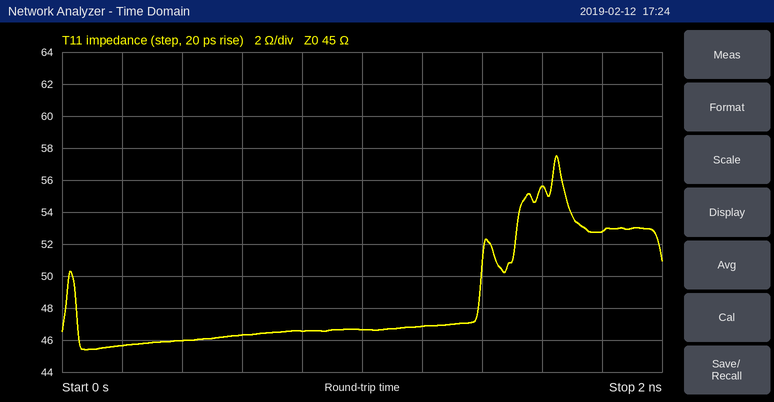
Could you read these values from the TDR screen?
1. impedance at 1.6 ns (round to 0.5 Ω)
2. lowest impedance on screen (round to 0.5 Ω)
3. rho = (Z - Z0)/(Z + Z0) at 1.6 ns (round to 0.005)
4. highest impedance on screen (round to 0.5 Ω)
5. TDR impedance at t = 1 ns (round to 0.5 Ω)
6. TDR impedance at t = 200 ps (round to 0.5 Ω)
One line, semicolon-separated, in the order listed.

55.5 Ω; 45.5 Ω; +0.105; 57.5 Ω; 46.5 Ω; 45.5 Ω
